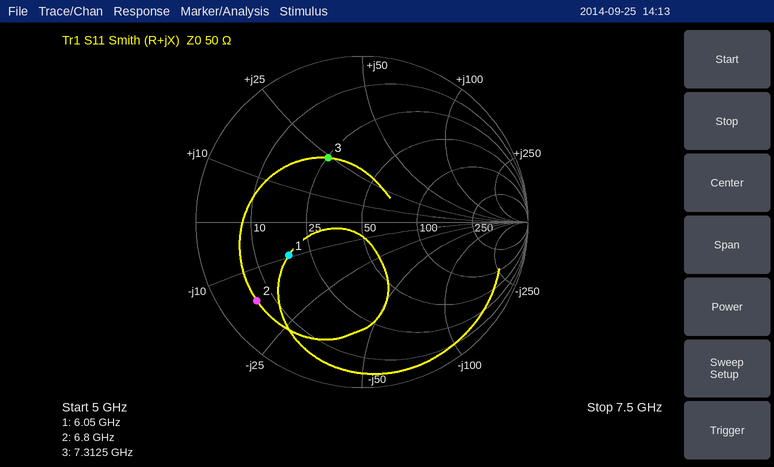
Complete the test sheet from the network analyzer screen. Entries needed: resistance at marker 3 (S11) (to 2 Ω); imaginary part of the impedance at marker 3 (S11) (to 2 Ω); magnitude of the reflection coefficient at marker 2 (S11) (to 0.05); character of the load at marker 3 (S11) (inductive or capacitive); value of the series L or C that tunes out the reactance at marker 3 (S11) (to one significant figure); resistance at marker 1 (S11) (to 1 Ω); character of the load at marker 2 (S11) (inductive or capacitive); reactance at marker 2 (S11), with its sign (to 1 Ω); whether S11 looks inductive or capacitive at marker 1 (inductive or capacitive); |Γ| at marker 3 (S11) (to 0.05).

26 Ω
+24 Ω
0.80
inductive
900 fF
18 Ω
capacitive
-16 Ω
capacitive
0.45
